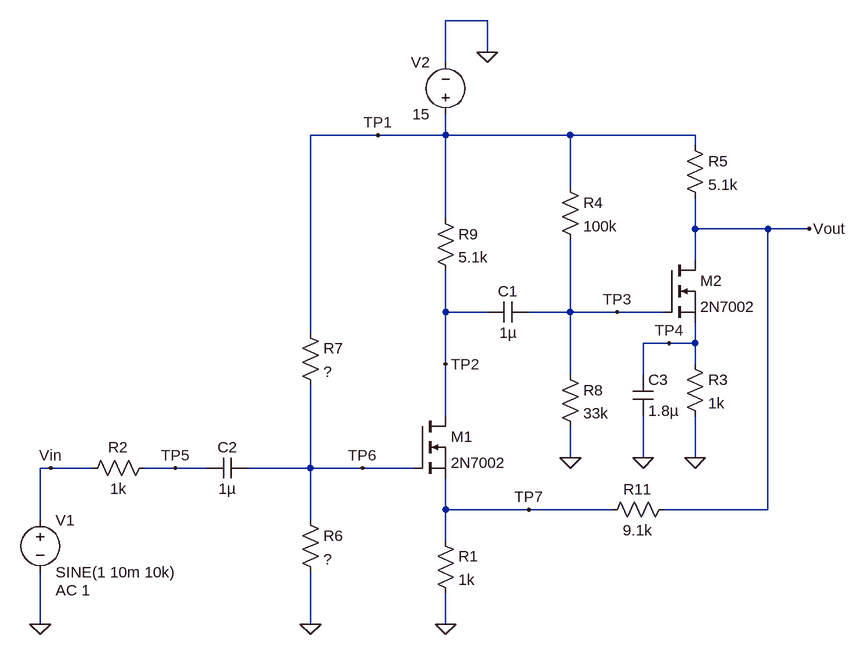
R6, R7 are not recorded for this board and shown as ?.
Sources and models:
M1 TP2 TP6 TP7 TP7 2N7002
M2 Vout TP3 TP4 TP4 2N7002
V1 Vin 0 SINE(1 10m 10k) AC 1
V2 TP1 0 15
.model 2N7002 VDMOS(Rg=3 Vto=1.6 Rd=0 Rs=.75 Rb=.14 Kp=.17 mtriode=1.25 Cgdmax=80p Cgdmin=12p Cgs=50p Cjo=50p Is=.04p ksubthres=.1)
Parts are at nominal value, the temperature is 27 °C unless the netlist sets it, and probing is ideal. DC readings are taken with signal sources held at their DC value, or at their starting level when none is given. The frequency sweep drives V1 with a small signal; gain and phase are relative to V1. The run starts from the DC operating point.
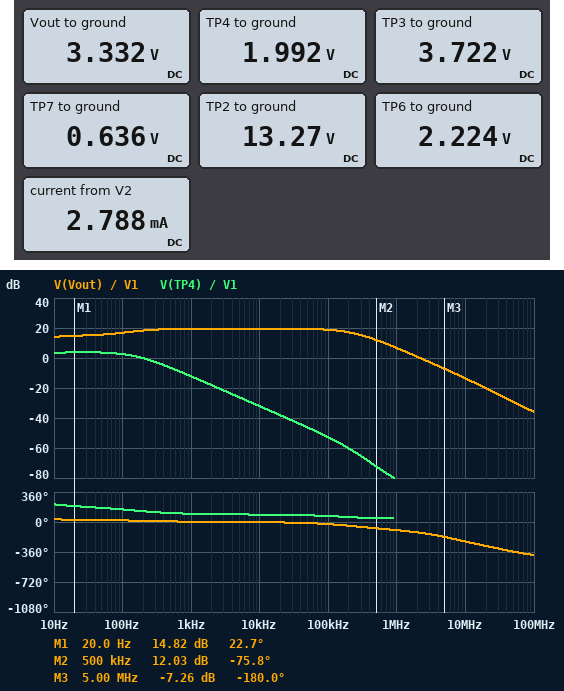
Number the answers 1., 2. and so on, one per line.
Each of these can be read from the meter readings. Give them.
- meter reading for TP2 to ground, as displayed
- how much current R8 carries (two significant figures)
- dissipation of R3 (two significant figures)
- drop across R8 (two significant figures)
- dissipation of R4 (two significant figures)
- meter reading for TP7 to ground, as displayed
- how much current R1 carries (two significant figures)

1. 13.27 V
2. 110 µA
3. 4.0 mW
4. 3.7 V
5. 1.3 mW
6. 0.636 V
7. 640 µA
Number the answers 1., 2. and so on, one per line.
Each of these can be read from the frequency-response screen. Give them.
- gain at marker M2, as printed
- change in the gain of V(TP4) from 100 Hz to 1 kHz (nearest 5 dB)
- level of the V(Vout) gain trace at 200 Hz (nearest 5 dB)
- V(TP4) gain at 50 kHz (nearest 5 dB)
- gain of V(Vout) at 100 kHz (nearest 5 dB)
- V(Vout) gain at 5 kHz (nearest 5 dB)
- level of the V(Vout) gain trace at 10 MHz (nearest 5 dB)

1. 12.03 dB
2. -15 dB
3. 20 dB
4. -45 dB
5. 20 dB
6. 20 dB
7. -15 dB
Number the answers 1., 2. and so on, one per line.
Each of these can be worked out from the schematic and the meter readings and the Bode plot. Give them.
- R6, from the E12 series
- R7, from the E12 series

1. 47 kΩ
2. 270 kΩ
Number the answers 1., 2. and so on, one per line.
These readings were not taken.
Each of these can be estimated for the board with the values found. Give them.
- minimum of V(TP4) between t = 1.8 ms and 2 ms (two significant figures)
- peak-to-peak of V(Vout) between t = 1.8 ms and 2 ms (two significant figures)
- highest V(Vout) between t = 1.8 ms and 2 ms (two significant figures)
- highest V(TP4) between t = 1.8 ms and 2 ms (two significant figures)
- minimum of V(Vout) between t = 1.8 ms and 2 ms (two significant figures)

1. 2.0 V
2. 190 mV
3. 3.4 V
4. 2.0 V
5. 3.2 V
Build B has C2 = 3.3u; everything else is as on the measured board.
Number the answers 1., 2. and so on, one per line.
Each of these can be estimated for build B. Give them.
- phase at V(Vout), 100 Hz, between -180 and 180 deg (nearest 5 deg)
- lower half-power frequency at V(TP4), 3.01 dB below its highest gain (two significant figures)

1. 15 deg
2. 2.8 Hz
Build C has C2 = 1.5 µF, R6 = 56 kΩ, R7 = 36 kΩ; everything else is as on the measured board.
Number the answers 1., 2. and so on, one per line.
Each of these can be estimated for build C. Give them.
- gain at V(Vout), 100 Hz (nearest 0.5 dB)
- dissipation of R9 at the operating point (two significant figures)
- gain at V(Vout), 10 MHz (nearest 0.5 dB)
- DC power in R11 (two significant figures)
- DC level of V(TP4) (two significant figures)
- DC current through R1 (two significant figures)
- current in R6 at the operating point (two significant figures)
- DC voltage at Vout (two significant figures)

1. -57.0 dB
2. 30 mW
3. -11.0 dB
4. 230 µW
5. 2.0 V
6. 2.6 mA
7. 160 µA
8. 4.0 V
